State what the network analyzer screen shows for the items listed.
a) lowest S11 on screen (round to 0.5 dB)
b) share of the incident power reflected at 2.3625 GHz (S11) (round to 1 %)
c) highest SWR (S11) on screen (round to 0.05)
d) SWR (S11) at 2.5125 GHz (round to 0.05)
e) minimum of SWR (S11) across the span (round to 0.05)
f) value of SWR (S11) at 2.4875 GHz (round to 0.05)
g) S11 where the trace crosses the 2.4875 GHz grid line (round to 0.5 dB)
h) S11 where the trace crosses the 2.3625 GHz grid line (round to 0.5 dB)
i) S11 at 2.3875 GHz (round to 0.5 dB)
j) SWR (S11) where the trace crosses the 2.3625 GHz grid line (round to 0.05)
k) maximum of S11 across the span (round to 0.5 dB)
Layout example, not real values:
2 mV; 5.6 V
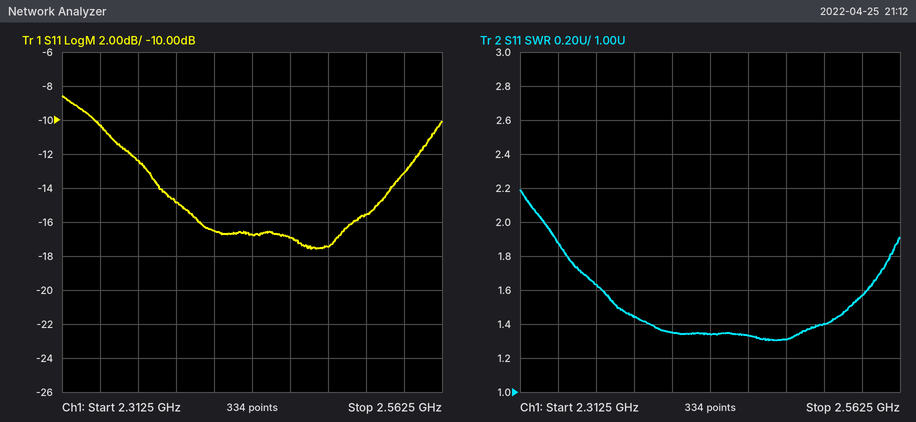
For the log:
-17.5 dB; 6 %; 2.20; 1.40; 1.30; 1.30; -17.5 dB; -12.5 dB; -15.0 dB; 1.65; -8.5 dB
